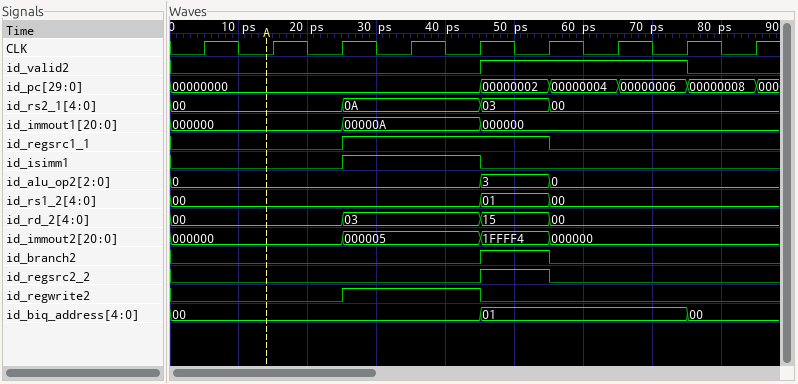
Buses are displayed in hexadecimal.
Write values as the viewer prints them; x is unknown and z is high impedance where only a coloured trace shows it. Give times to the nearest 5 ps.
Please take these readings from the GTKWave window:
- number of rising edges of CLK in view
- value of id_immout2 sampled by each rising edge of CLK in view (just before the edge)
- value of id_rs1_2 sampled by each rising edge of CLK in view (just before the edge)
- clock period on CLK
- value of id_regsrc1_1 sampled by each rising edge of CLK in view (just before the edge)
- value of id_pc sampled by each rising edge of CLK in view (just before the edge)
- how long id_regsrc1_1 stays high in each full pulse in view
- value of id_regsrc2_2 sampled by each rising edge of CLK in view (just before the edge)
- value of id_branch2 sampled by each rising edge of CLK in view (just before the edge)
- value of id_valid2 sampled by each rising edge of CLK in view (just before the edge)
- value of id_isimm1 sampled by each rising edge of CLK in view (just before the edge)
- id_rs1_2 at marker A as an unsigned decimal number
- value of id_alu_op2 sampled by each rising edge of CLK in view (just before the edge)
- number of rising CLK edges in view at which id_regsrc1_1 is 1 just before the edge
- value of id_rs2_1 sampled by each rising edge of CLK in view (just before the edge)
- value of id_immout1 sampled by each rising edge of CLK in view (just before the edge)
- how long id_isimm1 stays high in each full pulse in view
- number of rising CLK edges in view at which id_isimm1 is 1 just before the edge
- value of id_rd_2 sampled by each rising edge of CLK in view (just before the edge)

9
000000, 000000, 000000, 000005, 000005, 1FFFF4, 000000, 000000, 000000
00, 00, 00, 00, 00, 01, 00, 00, 00
10 ps
0 0 0 1 1 1 0 0 0
00000000, 00000000, 00000000, 00000000, 00000000, 00000002, 00000004, 00000006, 00000008
30 ps
0 0 0 0 0 1 0 0 0
0 0 0 0 0 1 0 0 0
0 0 0 0 0 1 1 1 0
0 0 0 1 1 0 0 0 0
0
0, 0, 0, 0, 0, 3, 0, 0, 0
3
00, 00, 00, 0A, 0A, 03, 00, 00, 00
000000, 000000, 000000, 00000A, 00000A, 000000, 000000, 000000, 000000
20 ps
2
00, 00, 00, 03, 03, 15, 00, 00, 00
